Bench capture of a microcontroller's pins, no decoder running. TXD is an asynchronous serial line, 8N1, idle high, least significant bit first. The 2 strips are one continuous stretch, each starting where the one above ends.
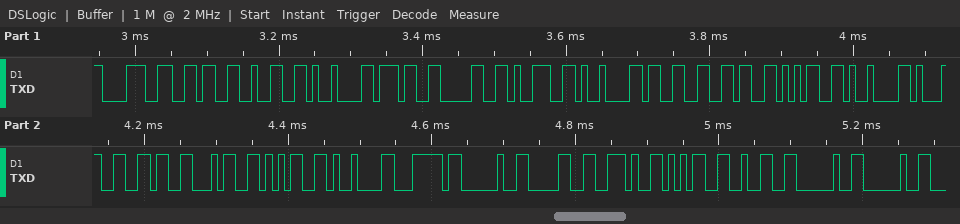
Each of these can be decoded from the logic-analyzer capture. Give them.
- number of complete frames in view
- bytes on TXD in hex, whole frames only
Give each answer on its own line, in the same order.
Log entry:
25
38 36 32 09 37 30 39 09 33 36 35 09 31 36 34 35 09 7C 20 30 2E 35 32 20 20
